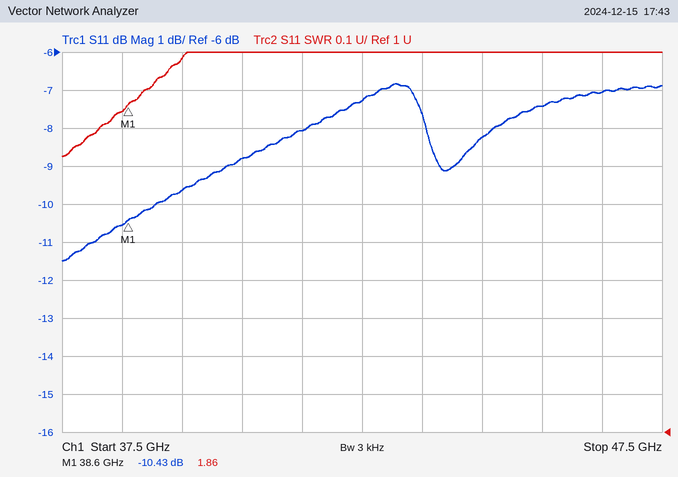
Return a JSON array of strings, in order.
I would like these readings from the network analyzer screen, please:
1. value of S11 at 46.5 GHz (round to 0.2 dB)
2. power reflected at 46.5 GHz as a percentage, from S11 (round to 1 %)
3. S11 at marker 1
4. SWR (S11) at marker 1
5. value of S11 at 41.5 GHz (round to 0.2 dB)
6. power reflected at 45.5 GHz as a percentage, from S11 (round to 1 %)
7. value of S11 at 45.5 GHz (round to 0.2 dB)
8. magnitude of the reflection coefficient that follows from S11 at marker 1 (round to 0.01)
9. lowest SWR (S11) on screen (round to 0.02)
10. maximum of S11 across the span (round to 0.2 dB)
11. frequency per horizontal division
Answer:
["-7.0 dB", "20 %", "-10.43 dB", "1.86", "-8.0 dB", "18 %", "-7.4 dB", "0.30", "1.72", "-6.8 dB", "1 GHz"]
